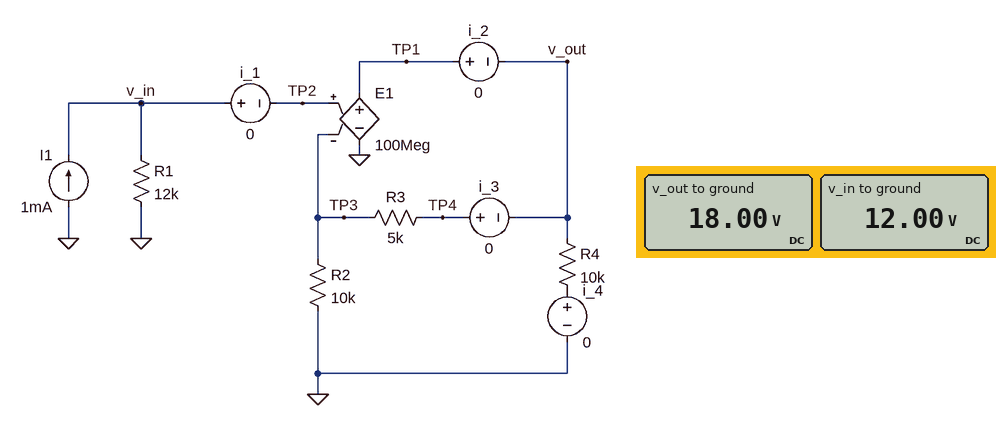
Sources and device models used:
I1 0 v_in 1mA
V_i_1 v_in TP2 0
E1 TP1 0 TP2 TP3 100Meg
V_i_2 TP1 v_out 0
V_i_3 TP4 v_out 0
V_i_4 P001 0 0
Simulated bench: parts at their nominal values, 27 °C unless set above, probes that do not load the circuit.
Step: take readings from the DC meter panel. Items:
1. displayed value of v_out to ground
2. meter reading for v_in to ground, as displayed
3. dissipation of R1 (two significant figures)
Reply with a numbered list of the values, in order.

1. 18.00 V
2. 12.00 V
3. 12 mW
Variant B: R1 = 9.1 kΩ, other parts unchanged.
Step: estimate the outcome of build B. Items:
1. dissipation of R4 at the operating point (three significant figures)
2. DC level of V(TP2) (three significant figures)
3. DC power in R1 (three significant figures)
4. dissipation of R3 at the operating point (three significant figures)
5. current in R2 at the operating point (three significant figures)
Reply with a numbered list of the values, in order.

1. 18.6 mW
2. 9.10 V
3. 9.10 mW
4. 4.14 mW
5. 910 µA
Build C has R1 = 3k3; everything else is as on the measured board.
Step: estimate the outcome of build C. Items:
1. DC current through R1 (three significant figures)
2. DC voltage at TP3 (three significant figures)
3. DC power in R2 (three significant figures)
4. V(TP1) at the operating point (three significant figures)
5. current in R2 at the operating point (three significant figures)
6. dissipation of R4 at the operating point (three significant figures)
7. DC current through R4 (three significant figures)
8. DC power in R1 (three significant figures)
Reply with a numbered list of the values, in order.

1. 1.00 mA
2. 3.30 V
3. 1.09 mW
4. 4.95 V
5. 330 µA
6. 2.45 mW
7. 495 µA
8. 3.30 mW
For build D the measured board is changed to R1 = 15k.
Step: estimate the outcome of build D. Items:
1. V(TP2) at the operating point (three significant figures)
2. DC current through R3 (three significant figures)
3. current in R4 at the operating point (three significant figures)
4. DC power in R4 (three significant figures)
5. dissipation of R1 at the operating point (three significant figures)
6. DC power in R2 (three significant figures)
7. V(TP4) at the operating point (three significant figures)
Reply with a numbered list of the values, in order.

1. 15.0 V
2. 1.50 mA
3. 2.25 mA
4. 50.6 mW
5. 15.0 mW
6. 22.5 mW
7. 22.5 V
